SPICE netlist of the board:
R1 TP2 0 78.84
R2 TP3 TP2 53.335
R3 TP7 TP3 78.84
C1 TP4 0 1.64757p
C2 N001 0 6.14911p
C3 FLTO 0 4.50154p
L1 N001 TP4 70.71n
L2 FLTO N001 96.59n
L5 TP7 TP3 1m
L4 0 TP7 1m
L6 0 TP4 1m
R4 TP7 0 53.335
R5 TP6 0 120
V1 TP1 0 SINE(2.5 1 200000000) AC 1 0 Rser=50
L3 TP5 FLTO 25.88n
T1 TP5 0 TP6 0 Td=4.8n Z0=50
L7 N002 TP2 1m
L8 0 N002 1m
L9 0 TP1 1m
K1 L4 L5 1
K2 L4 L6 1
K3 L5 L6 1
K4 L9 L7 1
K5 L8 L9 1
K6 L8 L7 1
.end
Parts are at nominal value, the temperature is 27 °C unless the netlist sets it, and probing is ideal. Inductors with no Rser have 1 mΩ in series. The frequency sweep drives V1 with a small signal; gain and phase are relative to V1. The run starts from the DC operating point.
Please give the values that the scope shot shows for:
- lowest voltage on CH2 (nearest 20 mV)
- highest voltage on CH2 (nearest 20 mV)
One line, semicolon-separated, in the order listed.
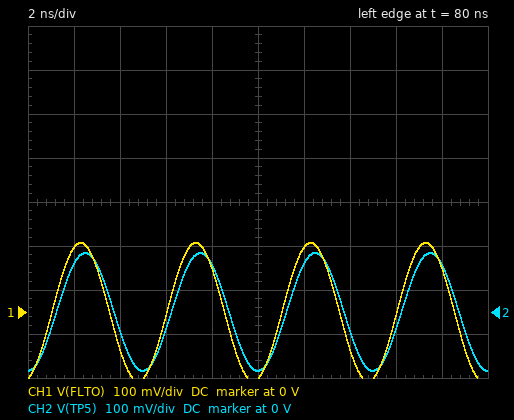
-140 mV; 140 mV
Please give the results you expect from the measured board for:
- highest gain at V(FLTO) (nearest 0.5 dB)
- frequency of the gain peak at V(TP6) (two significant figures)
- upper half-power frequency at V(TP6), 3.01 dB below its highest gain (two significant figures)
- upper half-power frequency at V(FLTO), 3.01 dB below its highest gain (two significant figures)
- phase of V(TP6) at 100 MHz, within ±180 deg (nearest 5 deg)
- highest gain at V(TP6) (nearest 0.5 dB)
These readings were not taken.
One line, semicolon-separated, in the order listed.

-11.0 dB; 280 MHz; 340 MHz; 300 MHz; 135 deg; -13.5 dB
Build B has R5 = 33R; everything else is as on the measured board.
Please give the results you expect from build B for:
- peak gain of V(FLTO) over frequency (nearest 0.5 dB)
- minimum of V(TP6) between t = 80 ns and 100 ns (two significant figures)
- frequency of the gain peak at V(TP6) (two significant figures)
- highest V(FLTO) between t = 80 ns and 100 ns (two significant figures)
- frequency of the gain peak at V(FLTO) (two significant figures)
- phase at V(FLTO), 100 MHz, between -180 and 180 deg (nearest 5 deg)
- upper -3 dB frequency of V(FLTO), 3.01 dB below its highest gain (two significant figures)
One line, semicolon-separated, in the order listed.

-15.0 dB; -42 mV; 300 MHz; 53 mV; 310 MHz; -55 deg; 350 MHz
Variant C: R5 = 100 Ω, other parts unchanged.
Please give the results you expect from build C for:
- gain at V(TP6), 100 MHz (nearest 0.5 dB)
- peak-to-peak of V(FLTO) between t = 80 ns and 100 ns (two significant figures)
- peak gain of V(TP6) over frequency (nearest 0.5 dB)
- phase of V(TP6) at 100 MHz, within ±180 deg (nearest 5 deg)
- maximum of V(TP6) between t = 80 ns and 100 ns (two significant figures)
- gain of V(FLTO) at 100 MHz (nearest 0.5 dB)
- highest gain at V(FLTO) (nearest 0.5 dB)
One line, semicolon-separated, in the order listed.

-19.5 dB; 270 mV; -14.5 dB; 130 deg; 120 mV; -19.0 dB; -12.0 dB
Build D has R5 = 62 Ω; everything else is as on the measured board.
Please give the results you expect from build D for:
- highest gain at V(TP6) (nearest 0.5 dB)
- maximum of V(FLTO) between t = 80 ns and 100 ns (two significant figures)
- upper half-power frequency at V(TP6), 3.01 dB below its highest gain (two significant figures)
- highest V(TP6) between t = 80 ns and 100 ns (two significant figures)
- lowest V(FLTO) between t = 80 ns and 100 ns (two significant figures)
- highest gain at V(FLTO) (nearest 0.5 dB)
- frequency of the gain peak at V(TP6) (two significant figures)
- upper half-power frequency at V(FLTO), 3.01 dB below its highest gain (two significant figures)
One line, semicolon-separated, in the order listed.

-17.0 dB; 89 mV; 340 MHz; 76 mV; -89 mV; -14.5 dB; 290 MHz; 330 MHz
